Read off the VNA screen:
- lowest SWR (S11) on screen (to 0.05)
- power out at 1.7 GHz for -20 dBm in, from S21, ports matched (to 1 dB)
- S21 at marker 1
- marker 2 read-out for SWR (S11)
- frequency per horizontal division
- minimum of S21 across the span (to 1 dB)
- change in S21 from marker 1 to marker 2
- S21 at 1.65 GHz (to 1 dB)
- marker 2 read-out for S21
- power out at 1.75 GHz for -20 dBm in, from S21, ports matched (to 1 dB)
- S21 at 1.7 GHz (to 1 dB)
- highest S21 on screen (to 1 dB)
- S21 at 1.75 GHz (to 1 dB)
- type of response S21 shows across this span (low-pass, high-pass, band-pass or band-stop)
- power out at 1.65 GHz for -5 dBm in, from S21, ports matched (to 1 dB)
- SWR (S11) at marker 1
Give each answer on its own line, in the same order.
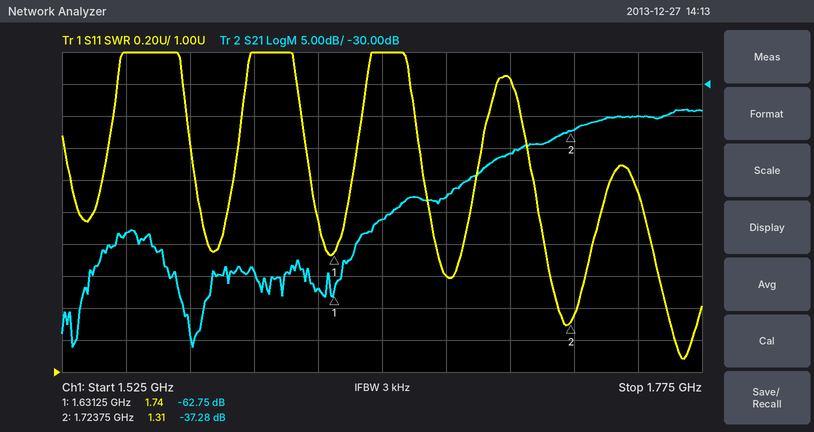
1.10
-61 dBm
-62.75 dB
1.31
25 MHz
-71 dB
25.47 dB
-51 dB
-37.28 dB
-55 dBm
-41 dB
-34 dB
-35 dB
high-pass
-56 dBm
1.74
